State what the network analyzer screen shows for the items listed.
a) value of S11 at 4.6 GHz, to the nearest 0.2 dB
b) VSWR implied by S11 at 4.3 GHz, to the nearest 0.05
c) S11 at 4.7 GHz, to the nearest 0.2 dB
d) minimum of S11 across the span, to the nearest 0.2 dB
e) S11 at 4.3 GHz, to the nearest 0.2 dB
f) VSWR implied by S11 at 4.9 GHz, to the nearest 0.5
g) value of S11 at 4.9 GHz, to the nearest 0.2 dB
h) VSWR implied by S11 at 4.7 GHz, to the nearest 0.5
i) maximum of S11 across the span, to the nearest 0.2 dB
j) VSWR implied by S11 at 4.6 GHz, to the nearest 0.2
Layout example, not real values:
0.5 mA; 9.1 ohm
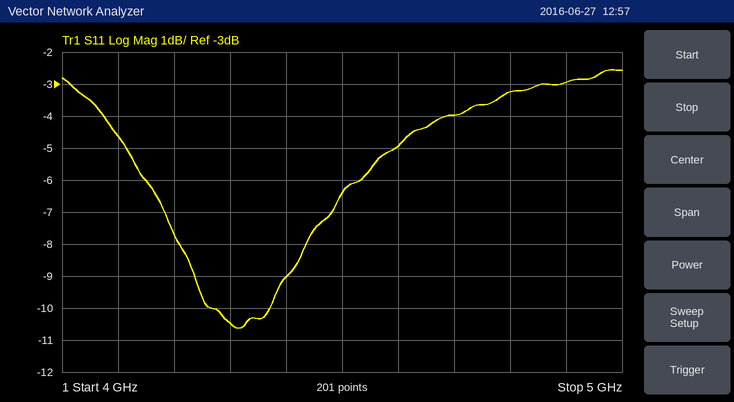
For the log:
-5.0 dB; 1.85; -4.0 dB; -10.6 dB; -10.4 dB; 6.0; -3.0 dB; 4.5; -2.6 dB; 3.6
